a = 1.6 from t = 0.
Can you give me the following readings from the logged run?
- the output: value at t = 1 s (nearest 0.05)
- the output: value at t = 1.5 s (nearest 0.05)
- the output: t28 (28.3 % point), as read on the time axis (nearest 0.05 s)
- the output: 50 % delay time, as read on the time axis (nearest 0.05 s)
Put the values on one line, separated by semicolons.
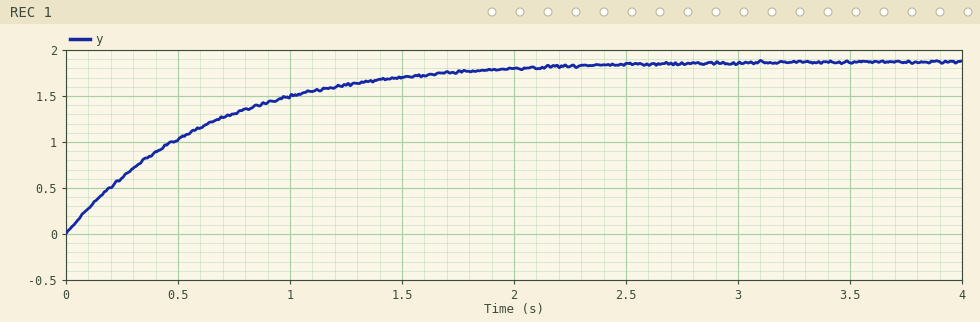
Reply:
1.50; 1.70; 0.20 s; 0.45 s
